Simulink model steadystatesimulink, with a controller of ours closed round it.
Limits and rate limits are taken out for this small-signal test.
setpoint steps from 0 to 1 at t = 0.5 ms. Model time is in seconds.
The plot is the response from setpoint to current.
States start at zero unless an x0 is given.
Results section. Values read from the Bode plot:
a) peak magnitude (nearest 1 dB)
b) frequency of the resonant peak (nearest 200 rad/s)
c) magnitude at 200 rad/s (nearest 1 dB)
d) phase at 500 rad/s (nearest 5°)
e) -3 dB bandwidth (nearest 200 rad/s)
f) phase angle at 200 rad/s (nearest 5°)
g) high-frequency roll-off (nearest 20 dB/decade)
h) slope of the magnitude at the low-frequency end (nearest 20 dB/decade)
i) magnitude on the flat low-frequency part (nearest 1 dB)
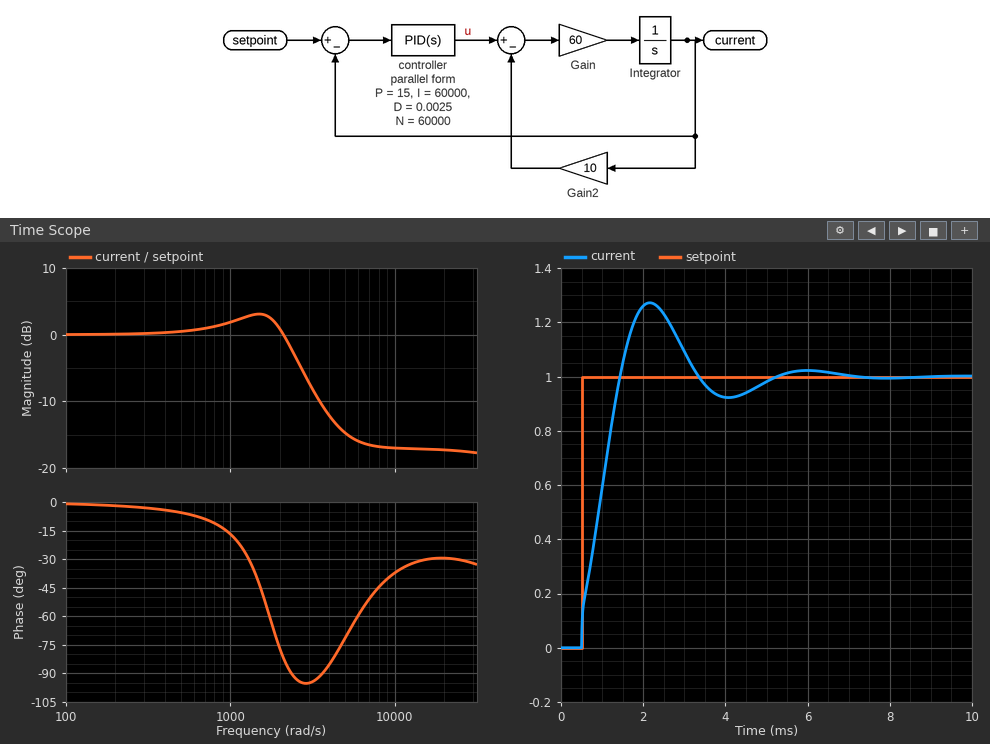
3 dB
1400 rad/s
0 dB
-5°
2400 rad/s
0°
0 dB/decade
0 dB/decade
0 dB
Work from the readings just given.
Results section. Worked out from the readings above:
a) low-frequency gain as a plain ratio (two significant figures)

1.0
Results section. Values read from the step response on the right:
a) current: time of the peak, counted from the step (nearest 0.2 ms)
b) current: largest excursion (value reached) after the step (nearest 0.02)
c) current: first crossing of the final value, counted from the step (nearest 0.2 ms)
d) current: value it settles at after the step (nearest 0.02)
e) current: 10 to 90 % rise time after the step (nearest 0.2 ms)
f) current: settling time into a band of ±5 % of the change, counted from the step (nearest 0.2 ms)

1.6 ms
1.28
1.0 ms
1.00
0.8 ms
4.2 ms
